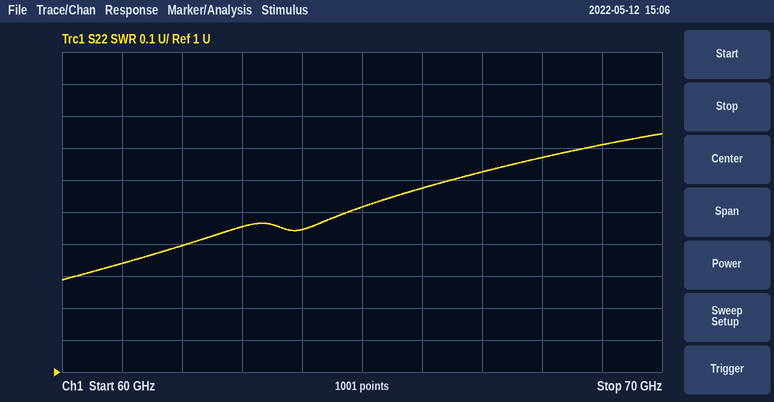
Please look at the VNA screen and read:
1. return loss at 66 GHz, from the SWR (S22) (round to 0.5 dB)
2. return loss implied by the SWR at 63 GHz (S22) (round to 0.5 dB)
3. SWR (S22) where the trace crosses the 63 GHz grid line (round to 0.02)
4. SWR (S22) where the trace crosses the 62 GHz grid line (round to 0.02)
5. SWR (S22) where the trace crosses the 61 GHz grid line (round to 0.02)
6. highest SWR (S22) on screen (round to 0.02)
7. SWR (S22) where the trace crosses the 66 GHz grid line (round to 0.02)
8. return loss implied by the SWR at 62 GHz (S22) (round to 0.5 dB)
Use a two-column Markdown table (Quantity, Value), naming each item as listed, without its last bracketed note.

| Quantity | Value |
|---|---|
| return loss at 66 GHz, from the SWR (S22) | 13.0 dB |
| return loss implied by the SWR at 63 GHz (S22) | 14.5 dB |
| SWR (S22) where the trace crosses the 63 GHz grid line | 1.46 |
| SWR (S22) where the trace crosses the 62 GHz grid line | 1.40 |
| SWR (S22) where the trace crosses the 61 GHz grid line | 1.34 |
| highest SWR (S22) on screen | 1.74 |
| SWR (S22) where the trace crosses the 66 GHz grid line | 1.58 |
| return loss implied by the SWR at 62 GHz (S22) | 15.5 dB |
